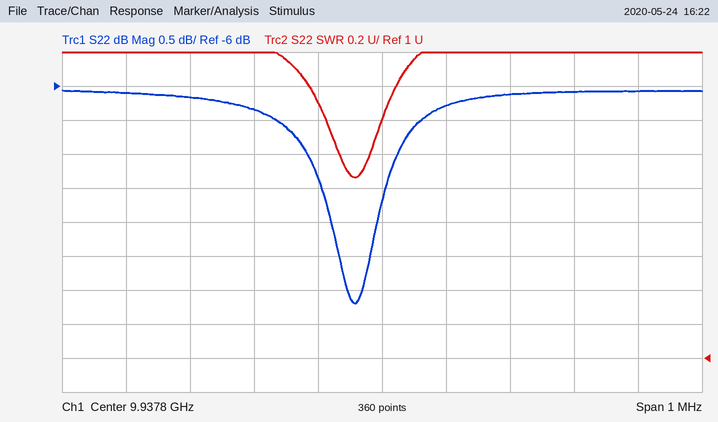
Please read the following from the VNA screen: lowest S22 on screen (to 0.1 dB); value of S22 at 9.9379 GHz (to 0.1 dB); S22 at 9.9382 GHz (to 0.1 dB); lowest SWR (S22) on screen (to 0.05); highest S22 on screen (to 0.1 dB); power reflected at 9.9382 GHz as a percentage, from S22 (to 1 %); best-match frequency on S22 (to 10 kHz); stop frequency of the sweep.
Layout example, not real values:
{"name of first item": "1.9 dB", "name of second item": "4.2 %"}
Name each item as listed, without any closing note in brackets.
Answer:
{"lowest S22 on screen": "-9.2 dB", "value of S22 at 9.9379 GHz": "-6.3 dB", "S22 at 9.9382 GHz": "-6.1 dB", "lowest SWR (S22) on screen": "2.05", "highest S22 on screen": "-6.1 dB", "power reflected at 9.9382 GHz as a percentage, from S22": "25 %", "best-match frequency on S22": "9.93776 GHz", "stop frequency of the sweep": "9.9383 GHz"}
